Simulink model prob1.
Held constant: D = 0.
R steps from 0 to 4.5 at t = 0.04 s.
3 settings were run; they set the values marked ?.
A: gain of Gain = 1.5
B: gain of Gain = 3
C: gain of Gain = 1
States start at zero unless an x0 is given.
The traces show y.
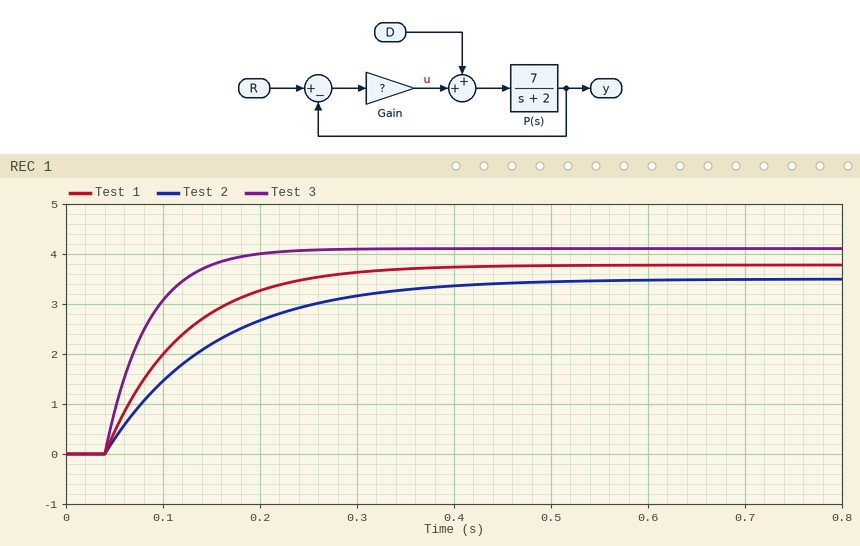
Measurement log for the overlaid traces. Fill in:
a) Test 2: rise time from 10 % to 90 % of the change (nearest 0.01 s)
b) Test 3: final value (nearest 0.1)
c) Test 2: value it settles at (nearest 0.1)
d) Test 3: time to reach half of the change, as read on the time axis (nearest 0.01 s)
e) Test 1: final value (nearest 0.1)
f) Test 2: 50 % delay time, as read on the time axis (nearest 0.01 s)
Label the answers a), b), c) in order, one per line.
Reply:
a) 0.24 s
b) 4.1
c) 3.5
d) 0.07 s
e) 3.8
f) 0.12 s
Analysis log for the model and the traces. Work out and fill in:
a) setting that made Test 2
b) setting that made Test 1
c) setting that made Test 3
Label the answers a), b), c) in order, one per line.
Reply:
a) C
b) A
c) B
